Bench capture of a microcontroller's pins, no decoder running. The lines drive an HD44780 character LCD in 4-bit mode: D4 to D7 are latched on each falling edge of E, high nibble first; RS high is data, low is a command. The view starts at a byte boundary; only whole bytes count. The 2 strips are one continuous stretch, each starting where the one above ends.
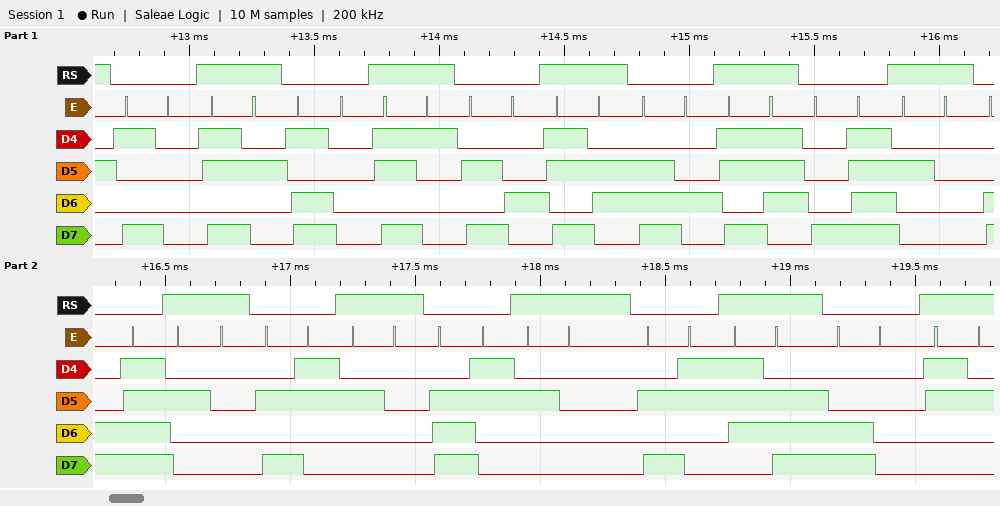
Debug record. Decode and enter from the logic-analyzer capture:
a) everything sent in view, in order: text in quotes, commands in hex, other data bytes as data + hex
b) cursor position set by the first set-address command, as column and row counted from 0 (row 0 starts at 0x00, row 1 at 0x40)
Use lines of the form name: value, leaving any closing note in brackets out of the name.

everything sent in view, in order: text in quotes, commands in hex, other data bytes as data + hex: 0x90 data B2 0xD0 data B1 0xA4 data B6 0xE4 data B7 0x8F " " 0xCF " " 0xA3 " " 0xE3 " " 0xA3 data 7E 0xC0 "2"
cursor position set by the first set-address command, as column and row counted from 0: column 16, row 0
